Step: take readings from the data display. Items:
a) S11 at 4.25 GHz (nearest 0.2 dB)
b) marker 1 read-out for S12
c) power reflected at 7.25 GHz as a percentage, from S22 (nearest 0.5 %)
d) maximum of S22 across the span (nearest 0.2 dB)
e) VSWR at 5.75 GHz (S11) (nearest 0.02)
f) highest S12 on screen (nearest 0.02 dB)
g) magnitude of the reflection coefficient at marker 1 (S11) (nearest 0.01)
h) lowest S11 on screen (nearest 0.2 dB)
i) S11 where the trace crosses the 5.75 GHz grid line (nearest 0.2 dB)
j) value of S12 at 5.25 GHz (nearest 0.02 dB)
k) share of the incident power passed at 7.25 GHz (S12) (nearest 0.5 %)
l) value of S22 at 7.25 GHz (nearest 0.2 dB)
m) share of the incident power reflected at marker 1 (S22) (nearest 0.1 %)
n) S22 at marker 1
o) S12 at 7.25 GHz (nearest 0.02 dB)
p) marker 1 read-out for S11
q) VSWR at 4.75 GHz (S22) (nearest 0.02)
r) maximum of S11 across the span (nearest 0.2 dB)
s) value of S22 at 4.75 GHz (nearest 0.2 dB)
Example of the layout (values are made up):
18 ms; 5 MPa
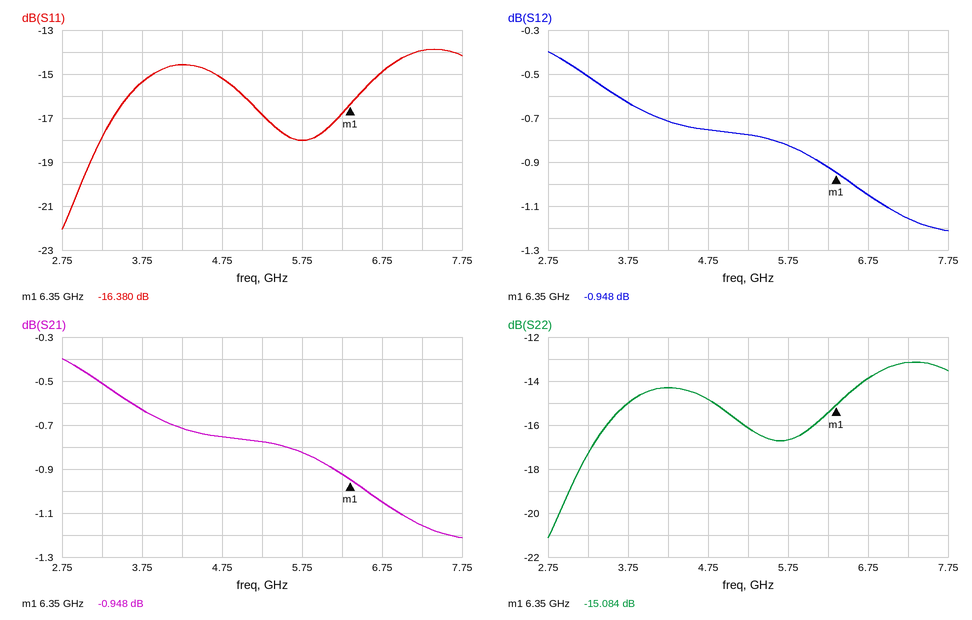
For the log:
-14.6 dB; -0.948 dB; 5.0 %; -13.2 dB; 1.28; -0.40 dB; 0.15; -22.0 dB; -18.0 dB; -0.78 dB; 76.5 %; -13.2 dB; 3.1 %; -15.084 dB; -1.16 dB; -16.380 dB; 1.44; -13.8 dB; -14.8 dB
